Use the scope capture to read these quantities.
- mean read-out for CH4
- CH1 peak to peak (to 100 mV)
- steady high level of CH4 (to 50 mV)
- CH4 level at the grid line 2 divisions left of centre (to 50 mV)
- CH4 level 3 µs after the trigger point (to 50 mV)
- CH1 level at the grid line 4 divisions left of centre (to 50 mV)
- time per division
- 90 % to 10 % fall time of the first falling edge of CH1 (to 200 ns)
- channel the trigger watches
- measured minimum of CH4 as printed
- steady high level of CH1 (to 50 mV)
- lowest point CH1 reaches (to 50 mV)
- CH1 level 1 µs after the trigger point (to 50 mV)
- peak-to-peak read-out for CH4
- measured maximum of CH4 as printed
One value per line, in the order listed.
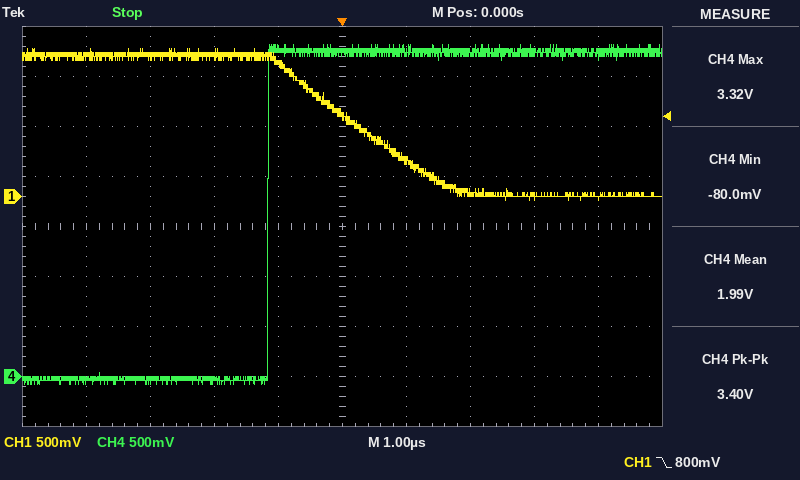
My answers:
1.99 V
1.50 V
3.25 V
-50 mV
3.25 V
1.40 V
1 µs
2.4 µs
CH1
-80.0 mV
1.40 V
-50 mV
350 mV
3.40 V
3.32 V
